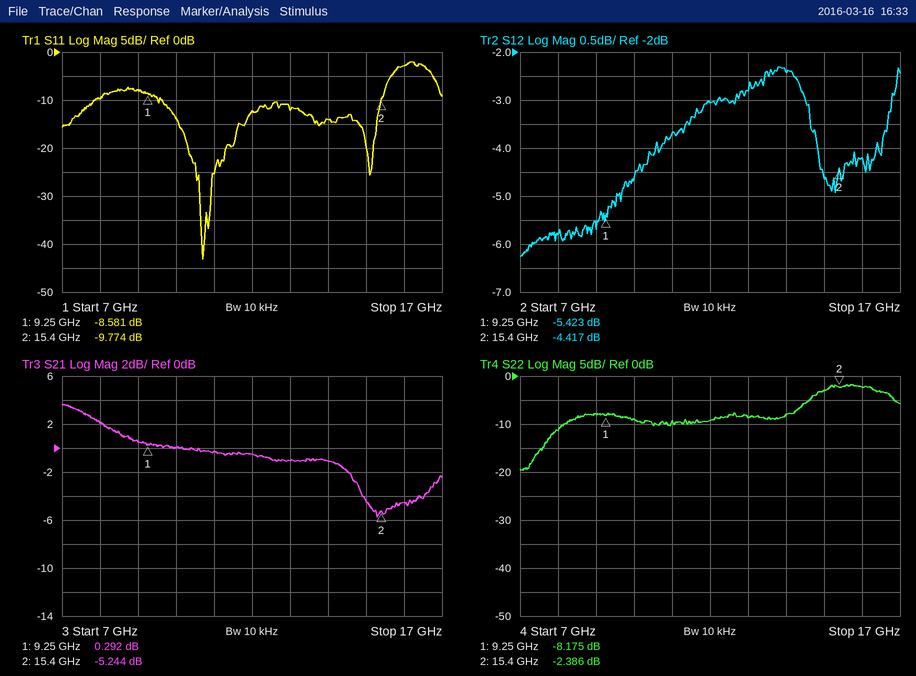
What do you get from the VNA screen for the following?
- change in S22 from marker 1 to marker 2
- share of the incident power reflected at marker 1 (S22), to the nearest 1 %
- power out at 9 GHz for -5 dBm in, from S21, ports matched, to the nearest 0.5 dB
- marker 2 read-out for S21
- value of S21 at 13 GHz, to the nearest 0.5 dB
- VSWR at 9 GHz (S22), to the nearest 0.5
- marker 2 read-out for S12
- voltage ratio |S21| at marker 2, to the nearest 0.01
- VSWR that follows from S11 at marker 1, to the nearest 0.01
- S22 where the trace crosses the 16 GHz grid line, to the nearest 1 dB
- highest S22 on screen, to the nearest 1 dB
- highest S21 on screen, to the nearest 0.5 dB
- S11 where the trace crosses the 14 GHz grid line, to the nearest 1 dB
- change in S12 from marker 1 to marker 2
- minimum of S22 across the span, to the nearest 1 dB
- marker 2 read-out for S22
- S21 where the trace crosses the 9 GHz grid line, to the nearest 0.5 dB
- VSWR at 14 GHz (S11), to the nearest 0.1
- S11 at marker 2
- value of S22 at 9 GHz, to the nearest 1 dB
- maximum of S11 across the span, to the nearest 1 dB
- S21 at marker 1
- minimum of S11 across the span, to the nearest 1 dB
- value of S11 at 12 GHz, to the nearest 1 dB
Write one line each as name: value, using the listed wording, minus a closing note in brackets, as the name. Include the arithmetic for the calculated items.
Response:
change in S22 from marker 1 to marker 2: -2.386 − (-8.175) = 5.789 dB
share of the incident power reflected at marker 1 (S22), to the nearest 1 %: 10^(-8.175/10) ≈ 15 %
power out at 9 GHz for -5 dBm in, from S21, ports matched, to the nearest 0.5 dB: -5 dBm + (0.5 dB) = -4.5 dBm
marker 2 read-out for S21: -5.244 dB
value of S21 at 13 GHz, to the nearest 0.5 dB: -1.0 dB
VSWR at 9 GHz (S22), to the nearest 0.5: |Γ| = 10^(-8/20) = 0.3981; VSWR = (1 + 0.3981)/(1 − 0.3981) ≈ 2.32, so 2.5 to the nearest 0.5
marker 2 read-out for S12: -4.417 dB
voltage ratio |S21| at marker 2, to the nearest 0.01: 10^(-5.244/20) ≈ 0.55
VSWR that follows from S11 at marker 1, to the nearest 0.01: (1 + 0.3723)/(1 − 0.3723) ≈ 2.19
S22 where the trace crosses the 16 GHz grid line, to the nearest 1 dB: -2 dB
highest S22 on screen, to the nearest 1 dB: -2 dB
highest S21 on screen, to the nearest 0.5 dB: 3.5 dB
S11 where the trace crosses the 14 GHz grid line, to the nearest 1 dB: -14 dB
change in S12 from marker 1 to marker 2: -4.417 − (-5.423) = 1.006 dB
minimum of S22 across the span, to the nearest 1 dB: -20 dB
marker 2 read-out for S22: -2.386 dB
S21 where the trace crosses the 9 GHz grid line, to the nearest 0.5 dB: 0.5 dB
VSWR at 14 GHz (S11), to the nearest 0.1: |Γ| = 10^(-14/20) = 0.1995; VSWR = (1 + 0.1995)/(1 − 0.1995) ≈ 1.5
S11 at marker 2: -9.774 dB
value of S22 at 9 GHz, to the nearest 1 dB: -8 dB
maximum of S11 across the span, to the nearest 1 dB: -2 dB
S21 at marker 1: 0.292 dB
minimum of S11 across the span, to the nearest 1 dB: -43 dB
value of S11 at 12 GHz, to the nearest 1 dB: -12 dB
